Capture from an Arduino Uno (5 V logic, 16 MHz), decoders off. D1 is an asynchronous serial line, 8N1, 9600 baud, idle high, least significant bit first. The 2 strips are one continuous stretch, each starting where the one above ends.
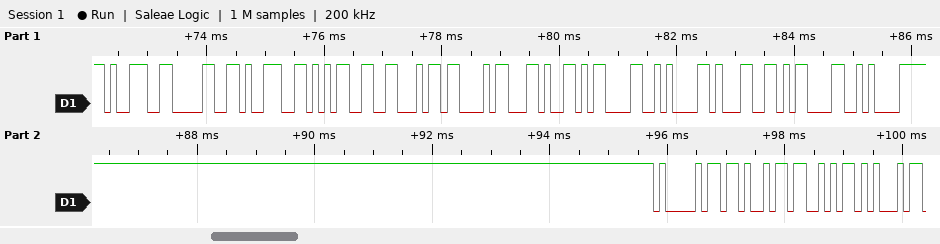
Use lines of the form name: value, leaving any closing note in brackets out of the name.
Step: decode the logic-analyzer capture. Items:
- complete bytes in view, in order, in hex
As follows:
complete bytes in view, in order, in hex: 0x39 0x30 0x39 0x35 0x46 0x43 0x2C 0x0D 0x0A 0x31 0x0D 0x0A 0x41 0x4B 0x53 0x45
